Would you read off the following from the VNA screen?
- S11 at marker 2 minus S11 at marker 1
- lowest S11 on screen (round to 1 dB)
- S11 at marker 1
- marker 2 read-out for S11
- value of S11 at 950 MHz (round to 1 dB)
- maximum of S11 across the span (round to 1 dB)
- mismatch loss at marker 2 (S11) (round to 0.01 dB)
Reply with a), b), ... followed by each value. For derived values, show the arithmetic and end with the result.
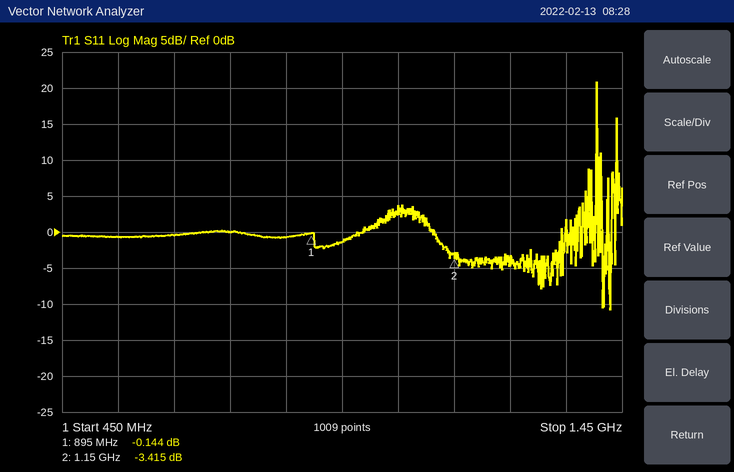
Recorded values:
a) -3.415 − (-0.144) = -3.271 dB
b) -11 dB
c) -0.144 dB
d) -3.415 dB
e) -1 dB
f) 21 dB
g) −10 log10(1 − 10^(-3.415/10)) ≈ 2.64 dB
